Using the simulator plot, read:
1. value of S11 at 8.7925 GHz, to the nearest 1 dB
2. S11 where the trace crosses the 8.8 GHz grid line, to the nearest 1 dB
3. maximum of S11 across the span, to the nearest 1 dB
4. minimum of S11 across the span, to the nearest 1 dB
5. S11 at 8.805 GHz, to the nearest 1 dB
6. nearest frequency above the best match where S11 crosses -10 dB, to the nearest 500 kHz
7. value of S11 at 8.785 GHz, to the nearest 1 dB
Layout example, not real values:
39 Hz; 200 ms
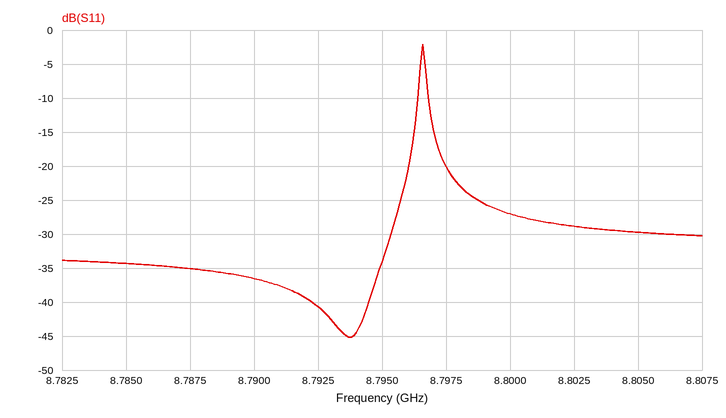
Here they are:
-41 dB; -27 dB; -2 dB; -45 dB; -30 dB; 8.7965 GHz; -34 dB
